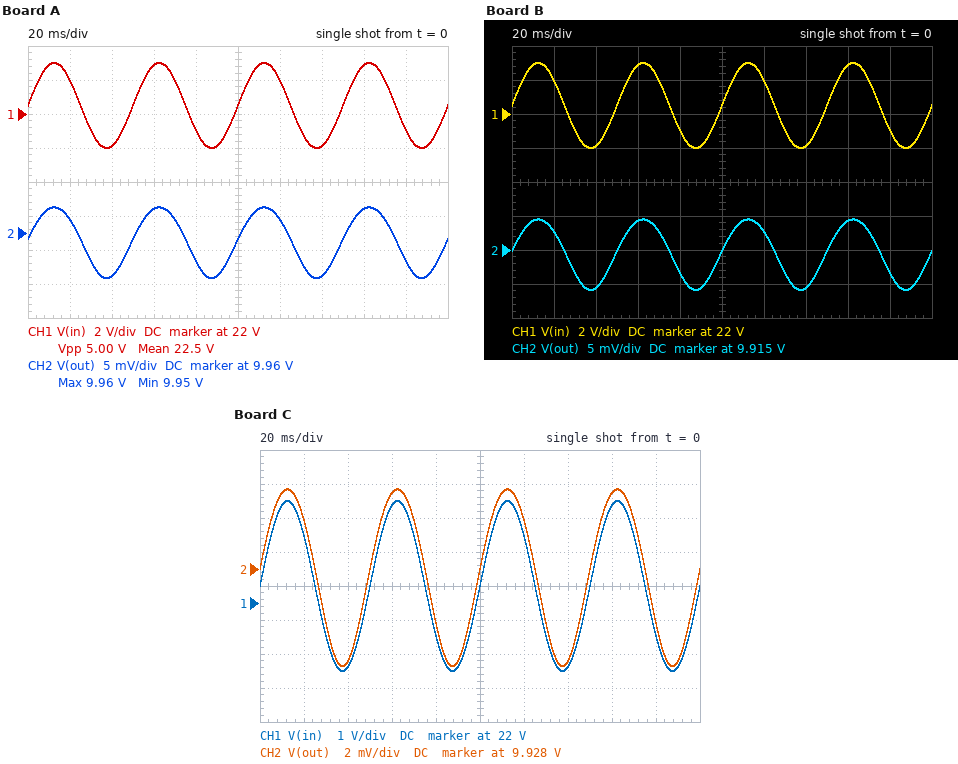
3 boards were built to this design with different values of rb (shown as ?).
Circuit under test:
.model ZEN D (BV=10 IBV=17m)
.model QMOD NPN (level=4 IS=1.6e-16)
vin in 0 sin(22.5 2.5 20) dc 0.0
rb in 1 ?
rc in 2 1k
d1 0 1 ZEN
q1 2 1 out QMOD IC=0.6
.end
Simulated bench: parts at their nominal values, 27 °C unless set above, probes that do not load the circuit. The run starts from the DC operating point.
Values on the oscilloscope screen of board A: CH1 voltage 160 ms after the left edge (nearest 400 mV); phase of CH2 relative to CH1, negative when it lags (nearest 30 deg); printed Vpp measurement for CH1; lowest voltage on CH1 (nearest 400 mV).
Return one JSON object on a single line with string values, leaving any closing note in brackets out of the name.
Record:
{"CH1 voltage 160 ms after the left edge": "24.8 V", "phase of CH2 relative to CH1, negative when it lags": "0 deg", "printed Vpp measurement for CH1": "5.00 V", "lowest voltage on CH1": "20.0 V"}
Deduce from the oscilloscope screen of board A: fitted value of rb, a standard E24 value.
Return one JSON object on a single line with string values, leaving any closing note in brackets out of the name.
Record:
{"fitted value of rb, a standard E24 value": "3.6 kΩ"}
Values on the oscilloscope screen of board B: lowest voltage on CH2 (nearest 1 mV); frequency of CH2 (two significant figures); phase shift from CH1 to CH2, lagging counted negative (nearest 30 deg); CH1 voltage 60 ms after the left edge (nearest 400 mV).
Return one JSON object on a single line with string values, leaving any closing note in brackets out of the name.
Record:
{"lowest voltage on CH2": "9.909 V", "frequency of CH2": "20 Hz", "phase shift from CH1 to CH2, lagging counted negative": "0 deg", "CH1 voltage 60 ms after the left edge": "24.8 V"}
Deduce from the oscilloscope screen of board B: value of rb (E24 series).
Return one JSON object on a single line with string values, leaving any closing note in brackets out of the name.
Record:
{"value of rb": "20 kΩ"}
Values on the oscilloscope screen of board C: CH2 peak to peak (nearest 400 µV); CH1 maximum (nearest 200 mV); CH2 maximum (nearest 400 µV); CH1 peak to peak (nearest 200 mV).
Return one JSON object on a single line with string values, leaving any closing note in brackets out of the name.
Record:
{"CH2 peak to peak": "10.4 mV", "CH1 maximum": "25.0 V", "CH2 maximum": "9.9328 V", "CH1 peak to peak": "5.0 V"}
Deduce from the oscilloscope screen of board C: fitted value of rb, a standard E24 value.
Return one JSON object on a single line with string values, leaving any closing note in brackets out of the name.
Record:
{"fitted value of rb, a standard E24 value": "12 kΩ"}
